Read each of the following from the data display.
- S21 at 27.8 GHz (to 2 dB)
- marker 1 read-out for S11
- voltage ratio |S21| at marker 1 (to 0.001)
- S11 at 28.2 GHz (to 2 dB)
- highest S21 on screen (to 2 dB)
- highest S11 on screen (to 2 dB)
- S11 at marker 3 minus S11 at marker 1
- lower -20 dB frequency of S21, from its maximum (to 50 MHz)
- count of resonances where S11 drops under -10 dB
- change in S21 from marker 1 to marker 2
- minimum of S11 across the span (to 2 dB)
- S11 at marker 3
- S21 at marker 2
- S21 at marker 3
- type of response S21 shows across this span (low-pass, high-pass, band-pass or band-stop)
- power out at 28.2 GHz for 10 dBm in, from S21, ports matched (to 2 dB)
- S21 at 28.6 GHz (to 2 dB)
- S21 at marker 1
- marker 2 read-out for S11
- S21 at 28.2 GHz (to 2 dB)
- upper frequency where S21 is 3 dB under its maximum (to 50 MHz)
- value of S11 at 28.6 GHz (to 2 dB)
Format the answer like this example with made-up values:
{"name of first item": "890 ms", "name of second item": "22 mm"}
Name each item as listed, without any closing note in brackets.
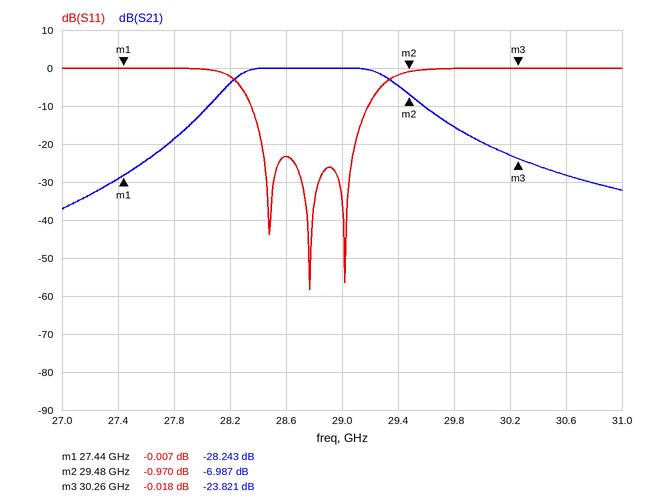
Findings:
{"S21 at 27.8 GHz": "-18 dB", "marker 1 read-out for S11": "-0.007 dB", "voltage ratio |S21| at marker 1": "0.039", "S11 at 28.2 GHz": "-2 dB", "highest S21 on screen": "0 dB", "highest S11 on screen": "0 dB", "S11 at marker 3 minus S11 at marker 1": "-0.011 dB", "lower -20 dB frequency of S21, from its maximum": "27.75 GHz", "count of resonances where S11 drops under -10 dB": "3", "change in S21 from marker 1 to marker 2": "21.256 dB", "minimum of S11 across the span": "-58 dB", "S11 at marker 3": "-0.018 dB", "S21 at marker 2": "-6.987 dB", "S21 at marker 3": "-23.821 dB", "type of response S21 shows across this span": "band-pass", "power out at 28.2 GHz for 10 dBm in, from S21, ports matched": "6 dBm", "S21 at 28.6 GHz": "0 dB", "S21 at marker 1": "-28.243 dB", "marker 2 read-out for S11": "-0.970 dB", "S21 at 28.2 GHz": "-4 dB", "upper frequency where S21 is 3 dB under its maximum": "29.35 GHz", "value of S11 at 28.6 GHz": "-24 dB"}
